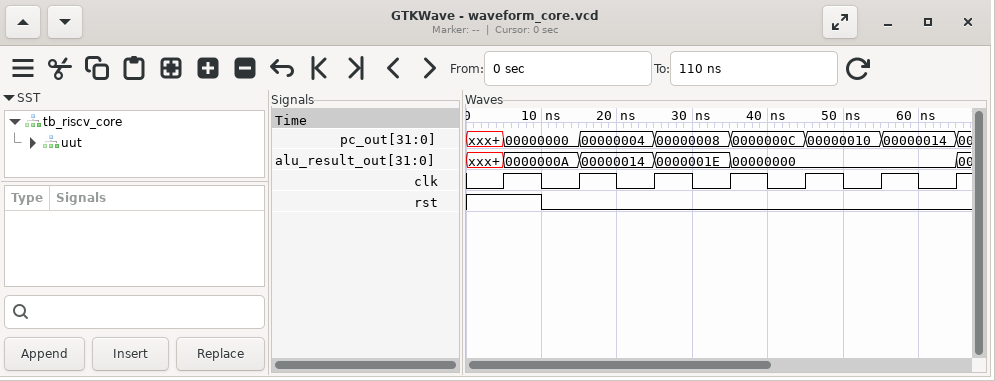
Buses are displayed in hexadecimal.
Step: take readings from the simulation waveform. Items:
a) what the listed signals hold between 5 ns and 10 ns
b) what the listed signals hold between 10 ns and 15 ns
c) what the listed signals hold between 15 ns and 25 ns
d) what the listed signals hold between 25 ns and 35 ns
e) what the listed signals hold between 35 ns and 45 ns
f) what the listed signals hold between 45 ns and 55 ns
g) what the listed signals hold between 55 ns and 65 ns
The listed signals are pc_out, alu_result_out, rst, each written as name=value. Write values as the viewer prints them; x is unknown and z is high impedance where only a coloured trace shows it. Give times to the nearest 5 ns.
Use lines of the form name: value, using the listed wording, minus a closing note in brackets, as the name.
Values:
what the listed signals hold between 5 ns and 10 ns: pc_out=00000000, alu_result_out=0000000A, rst=1
what the listed signals hold between 10 ns and 15 ns: pc_out=00000000, alu_result_out=0000000A, rst=0
what the listed signals hold between 15 ns and 25 ns: pc_out=00000004, alu_result_out=00000014, rst=0
what the listed signals hold between 25 ns and 35 ns: pc_out=00000008, alu_result_out=0000001E, rst=0
what the listed signals hold between 35 ns and 45 ns: pc_out=0000000C, alu_result_out=00000000, rst=0
what the listed signals hold between 45 ns and 55 ns: pc_out=00000010, alu_result_out=00000000, rst=0
what the listed signals hold between 55 ns and 65 ns: pc_out=00000014, alu_result_out=00000000, rst=0
